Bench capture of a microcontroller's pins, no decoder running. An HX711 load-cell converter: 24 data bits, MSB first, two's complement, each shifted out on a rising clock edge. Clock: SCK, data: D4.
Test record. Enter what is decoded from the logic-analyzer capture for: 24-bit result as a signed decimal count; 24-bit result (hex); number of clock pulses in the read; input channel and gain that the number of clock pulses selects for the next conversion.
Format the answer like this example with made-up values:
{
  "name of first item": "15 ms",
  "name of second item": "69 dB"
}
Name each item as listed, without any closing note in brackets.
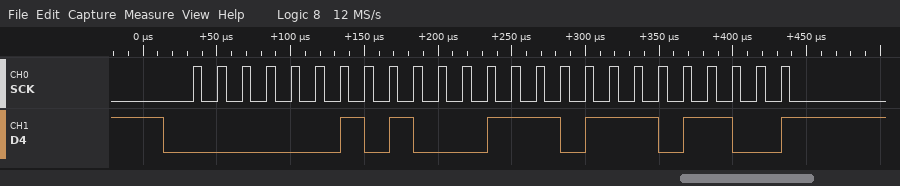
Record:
{
  "24-bit result as a signed decimal count": "167660",
  "24-bit result": "0x028EEC",
  "number of clock pulses in the read": "25",
  "input channel and gain that the number of clock pulses selects for the next conversion": "channel A, gain 128"
}
